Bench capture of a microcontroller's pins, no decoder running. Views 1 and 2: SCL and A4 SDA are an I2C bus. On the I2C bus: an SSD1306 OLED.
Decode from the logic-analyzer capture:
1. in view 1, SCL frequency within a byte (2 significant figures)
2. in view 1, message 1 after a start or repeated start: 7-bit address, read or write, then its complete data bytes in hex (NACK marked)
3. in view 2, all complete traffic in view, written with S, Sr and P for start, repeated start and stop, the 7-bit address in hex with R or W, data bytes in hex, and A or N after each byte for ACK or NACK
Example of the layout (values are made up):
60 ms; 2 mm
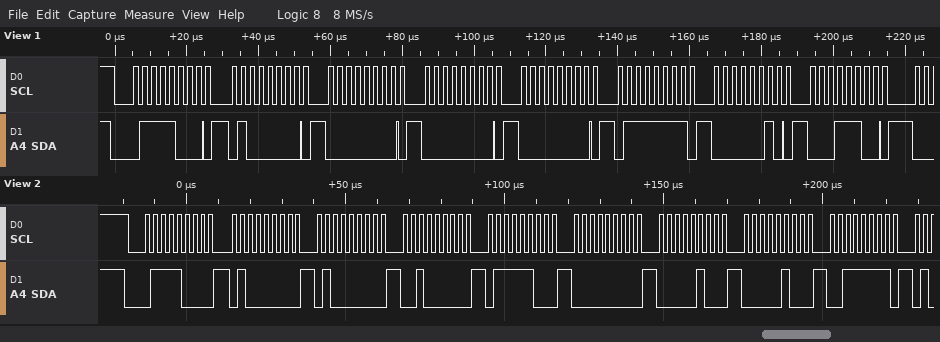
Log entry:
400 kHz; 0x3C write: 40 00 00 00 7F 02 1C; S 3CW A 40 A 40 A 20 A 7C A 00 A 04 A 04 A 3F A
